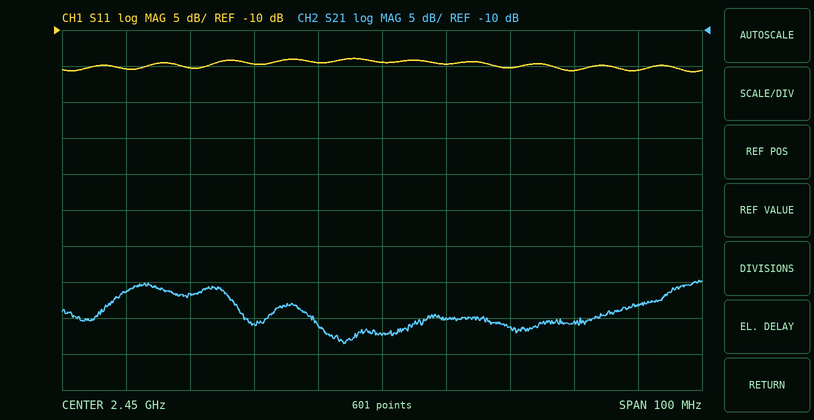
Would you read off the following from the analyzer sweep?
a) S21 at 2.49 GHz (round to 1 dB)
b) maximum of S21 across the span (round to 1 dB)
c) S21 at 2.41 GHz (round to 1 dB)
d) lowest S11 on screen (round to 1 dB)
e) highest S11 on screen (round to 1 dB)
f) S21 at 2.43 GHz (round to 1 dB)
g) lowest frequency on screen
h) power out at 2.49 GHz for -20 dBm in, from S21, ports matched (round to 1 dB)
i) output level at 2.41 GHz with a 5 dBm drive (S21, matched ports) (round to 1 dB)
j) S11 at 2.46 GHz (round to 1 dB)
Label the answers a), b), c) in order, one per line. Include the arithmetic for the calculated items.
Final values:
a) -48 dB
b) -45 dB
c) -46 dB
d) -16 dB
e) -14 dB
f) -51 dB
g) 2.4 GHz
h) -20 dBm + (-48 dB) = -68 dBm
i) 5 dBm + (-46 dB) = -41 dBm
j) -15 dB
